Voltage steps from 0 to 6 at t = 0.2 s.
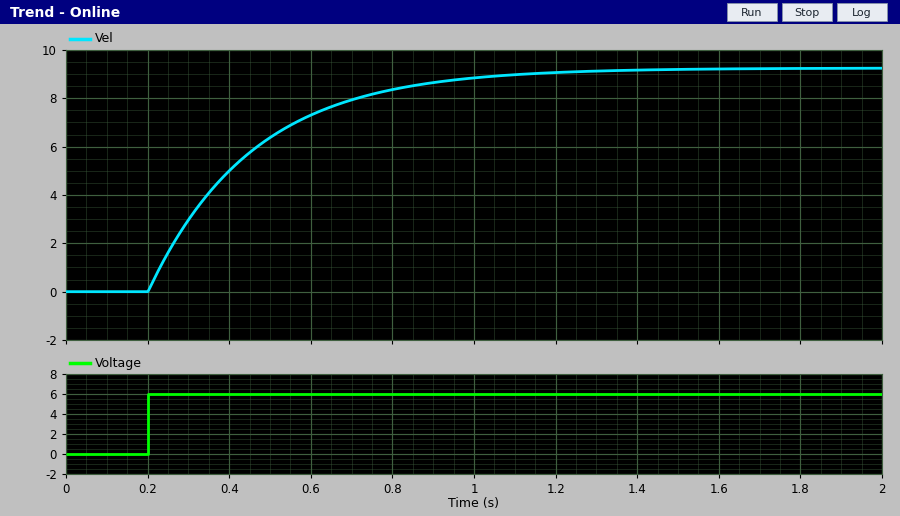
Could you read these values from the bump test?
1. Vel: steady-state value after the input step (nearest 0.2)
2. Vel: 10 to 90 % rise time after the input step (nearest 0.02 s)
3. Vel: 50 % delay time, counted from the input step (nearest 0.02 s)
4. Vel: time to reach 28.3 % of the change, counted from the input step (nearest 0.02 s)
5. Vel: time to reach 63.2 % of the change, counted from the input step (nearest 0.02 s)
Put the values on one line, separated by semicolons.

9.2; 0.56 s; 0.18 s; 0.08 s; 0.26 s
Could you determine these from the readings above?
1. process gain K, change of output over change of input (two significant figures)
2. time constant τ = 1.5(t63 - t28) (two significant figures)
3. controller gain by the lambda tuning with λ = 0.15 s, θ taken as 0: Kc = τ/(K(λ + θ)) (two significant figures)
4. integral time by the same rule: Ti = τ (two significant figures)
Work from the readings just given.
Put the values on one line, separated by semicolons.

1.5; 0.27 s; 1.2; 0.27 s
